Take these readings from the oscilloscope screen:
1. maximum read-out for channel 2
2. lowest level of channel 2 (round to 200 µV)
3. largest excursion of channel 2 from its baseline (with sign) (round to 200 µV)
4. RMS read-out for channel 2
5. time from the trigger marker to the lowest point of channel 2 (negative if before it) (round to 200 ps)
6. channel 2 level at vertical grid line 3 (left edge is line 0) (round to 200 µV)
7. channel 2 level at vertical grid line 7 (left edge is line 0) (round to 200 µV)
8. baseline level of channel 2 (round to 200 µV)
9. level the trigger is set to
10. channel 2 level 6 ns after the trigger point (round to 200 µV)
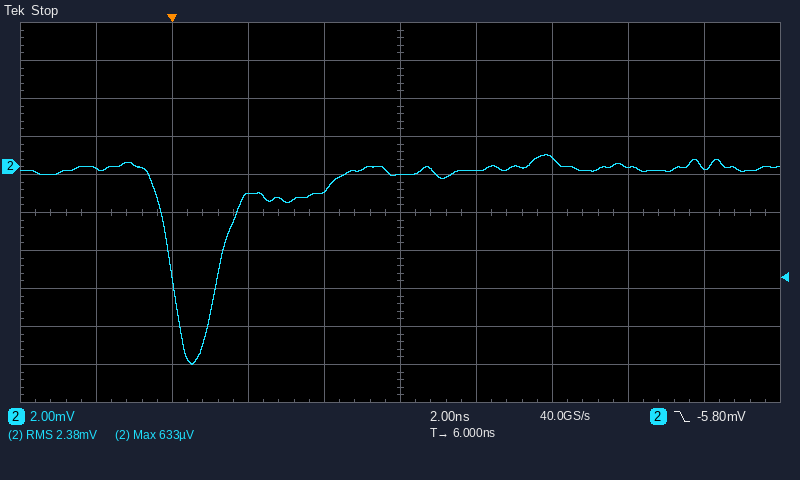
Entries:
633 µV
-10.4 mV
-10.2 mV
2.38 mV
+600 ps
-1.4 mV
400 µV
-200 µV
-5.80 mV
-400 µV
